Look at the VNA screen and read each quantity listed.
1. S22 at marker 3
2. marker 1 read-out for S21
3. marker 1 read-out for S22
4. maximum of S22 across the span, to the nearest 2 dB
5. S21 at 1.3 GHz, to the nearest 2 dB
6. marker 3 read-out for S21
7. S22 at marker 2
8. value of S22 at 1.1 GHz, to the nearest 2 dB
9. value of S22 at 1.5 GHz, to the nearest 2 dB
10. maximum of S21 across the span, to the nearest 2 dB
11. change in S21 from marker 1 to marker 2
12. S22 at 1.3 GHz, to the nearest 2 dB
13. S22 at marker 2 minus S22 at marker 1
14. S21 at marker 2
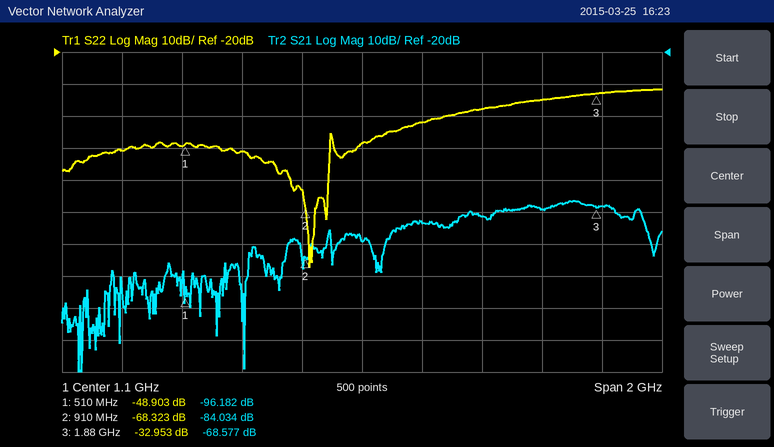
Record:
-32.953 dB
-96.182 dB
-48.903 dB
-32 dB
-74 dB
-68.577 dB
-68.323 dB
-48 dB
-38 dB
-66 dB
12.148 dB
-42 dB
-19.420 dB
-84.034 dB
